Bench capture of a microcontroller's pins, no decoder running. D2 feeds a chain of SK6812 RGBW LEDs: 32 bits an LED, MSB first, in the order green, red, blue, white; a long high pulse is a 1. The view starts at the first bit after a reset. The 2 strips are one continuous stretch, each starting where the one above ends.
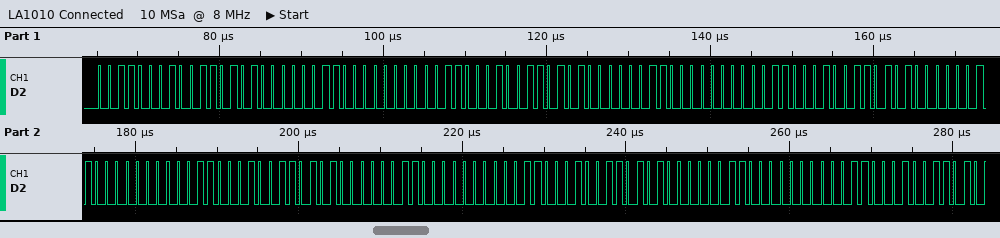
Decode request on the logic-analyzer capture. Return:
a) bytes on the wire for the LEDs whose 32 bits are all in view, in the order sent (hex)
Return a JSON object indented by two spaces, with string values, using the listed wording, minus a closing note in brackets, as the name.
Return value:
{
  "bytes on the wire for the LEDs whose 32 bits are all in view, in the order sent": "31 35 03 00 31 35 03 00 31 35 03 00 31 35 03 00 31 35 03 00"
}
